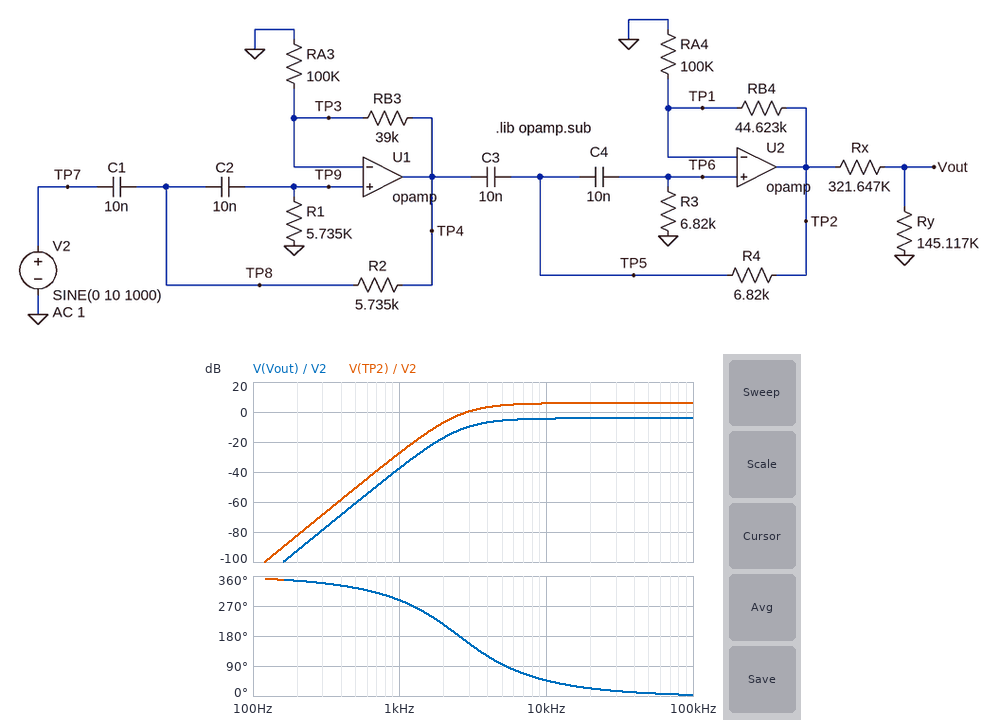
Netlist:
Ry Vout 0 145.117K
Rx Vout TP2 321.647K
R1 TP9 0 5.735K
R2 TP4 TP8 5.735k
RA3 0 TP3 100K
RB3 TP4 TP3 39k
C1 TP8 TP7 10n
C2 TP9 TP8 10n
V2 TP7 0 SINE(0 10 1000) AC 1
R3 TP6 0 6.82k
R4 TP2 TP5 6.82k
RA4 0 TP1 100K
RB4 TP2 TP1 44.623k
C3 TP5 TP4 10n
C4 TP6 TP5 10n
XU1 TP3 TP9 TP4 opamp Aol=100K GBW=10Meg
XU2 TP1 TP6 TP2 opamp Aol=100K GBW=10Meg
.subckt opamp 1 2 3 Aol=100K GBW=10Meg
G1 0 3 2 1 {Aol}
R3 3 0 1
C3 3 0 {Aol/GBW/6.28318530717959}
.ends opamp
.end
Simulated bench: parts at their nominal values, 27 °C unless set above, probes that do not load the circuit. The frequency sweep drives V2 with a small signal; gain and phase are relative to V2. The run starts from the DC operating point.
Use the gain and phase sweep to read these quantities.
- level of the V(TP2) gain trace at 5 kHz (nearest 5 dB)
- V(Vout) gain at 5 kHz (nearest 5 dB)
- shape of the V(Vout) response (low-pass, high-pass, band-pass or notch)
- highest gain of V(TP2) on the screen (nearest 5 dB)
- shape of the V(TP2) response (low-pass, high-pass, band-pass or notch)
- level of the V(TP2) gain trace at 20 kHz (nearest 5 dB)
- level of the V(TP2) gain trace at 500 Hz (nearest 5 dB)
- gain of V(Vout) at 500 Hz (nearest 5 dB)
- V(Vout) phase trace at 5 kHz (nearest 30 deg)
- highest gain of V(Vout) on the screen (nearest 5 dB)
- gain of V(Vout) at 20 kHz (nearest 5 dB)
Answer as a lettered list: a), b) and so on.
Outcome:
a) 5 dB
b) -5 dB
c) high-pass
d) 5 dB
e) high-pass
f) 5 dB
g) -50 dB
h) -60 dB
i) 90 deg
j) -5 dB
k) -5 dB
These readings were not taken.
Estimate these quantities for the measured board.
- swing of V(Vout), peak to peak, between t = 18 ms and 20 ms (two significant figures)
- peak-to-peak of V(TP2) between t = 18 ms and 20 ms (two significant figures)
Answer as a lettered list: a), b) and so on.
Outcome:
a) 270 mV
b) 870 mV
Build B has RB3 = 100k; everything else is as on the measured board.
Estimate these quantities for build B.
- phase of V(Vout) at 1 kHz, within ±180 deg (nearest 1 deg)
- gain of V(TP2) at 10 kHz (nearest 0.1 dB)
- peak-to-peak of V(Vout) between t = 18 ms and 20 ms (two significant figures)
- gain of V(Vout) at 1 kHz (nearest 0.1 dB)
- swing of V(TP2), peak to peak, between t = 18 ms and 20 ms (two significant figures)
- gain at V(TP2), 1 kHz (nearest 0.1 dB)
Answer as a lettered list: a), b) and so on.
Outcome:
a) -62 deg
b) 9.4 dB
c) 430 mV
d) -33.3 dB
e) 1.4 V
f) -23.2 dB
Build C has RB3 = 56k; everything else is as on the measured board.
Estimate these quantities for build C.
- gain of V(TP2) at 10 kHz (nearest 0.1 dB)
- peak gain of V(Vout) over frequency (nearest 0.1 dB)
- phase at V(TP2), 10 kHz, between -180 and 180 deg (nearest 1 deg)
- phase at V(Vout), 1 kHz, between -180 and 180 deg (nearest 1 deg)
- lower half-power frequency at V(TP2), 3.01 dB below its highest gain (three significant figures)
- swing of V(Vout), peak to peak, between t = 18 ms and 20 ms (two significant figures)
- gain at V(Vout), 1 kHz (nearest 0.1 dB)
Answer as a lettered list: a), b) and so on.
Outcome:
a) 6.9 dB
b) -3.1 dB
c) 44 deg
d) -70 deg
e) 3.49 kHz
f) 310 mV
g) -36.1 dB
